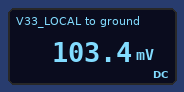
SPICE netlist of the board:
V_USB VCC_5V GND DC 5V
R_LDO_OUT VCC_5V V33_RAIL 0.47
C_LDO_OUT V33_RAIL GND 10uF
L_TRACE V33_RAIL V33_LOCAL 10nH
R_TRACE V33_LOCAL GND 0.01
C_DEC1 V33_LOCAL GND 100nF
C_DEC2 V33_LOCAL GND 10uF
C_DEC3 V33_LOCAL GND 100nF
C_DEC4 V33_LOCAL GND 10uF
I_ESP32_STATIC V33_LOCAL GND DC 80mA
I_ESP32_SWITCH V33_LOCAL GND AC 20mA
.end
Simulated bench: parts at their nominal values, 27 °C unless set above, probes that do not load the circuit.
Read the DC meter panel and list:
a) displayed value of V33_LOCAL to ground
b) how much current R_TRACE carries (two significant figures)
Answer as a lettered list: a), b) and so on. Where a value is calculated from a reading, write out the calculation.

a) 103.4 mV
b) (103.4 mV) / 10 mΩ = 10 A
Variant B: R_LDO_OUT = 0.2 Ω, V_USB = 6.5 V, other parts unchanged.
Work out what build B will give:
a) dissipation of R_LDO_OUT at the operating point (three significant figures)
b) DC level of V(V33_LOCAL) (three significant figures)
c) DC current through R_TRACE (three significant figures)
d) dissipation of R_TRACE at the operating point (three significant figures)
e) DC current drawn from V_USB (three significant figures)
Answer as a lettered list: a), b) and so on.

a) 192 W
b) 309 mV
c) 30.9 A
d) 9.53 W
e) 31.0 A
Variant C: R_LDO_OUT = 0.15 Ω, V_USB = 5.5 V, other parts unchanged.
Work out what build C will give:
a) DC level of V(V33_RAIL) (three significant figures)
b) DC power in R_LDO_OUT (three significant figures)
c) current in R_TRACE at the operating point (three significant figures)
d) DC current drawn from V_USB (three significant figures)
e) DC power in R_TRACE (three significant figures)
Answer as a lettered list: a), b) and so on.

a) 343 mV
b) 177 W
c) 34.3 A
d) 34.4 A
e) 11.8 W
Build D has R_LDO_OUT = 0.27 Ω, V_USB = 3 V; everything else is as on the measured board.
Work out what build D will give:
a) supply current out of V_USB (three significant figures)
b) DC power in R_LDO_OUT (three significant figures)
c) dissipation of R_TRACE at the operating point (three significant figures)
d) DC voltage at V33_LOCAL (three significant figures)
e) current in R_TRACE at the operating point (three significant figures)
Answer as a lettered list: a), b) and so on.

a) 10.7 A
b) 31.0 W
c) 1.13 W
d) 106 mV
e) 10.6 A
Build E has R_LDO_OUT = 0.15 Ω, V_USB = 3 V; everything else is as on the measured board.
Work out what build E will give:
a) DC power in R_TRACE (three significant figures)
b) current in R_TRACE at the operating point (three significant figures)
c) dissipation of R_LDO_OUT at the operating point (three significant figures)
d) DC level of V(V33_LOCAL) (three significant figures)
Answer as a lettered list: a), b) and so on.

a) 3.49 W
b) 18.7 A
c) 52.8 W
d) 187 mV
